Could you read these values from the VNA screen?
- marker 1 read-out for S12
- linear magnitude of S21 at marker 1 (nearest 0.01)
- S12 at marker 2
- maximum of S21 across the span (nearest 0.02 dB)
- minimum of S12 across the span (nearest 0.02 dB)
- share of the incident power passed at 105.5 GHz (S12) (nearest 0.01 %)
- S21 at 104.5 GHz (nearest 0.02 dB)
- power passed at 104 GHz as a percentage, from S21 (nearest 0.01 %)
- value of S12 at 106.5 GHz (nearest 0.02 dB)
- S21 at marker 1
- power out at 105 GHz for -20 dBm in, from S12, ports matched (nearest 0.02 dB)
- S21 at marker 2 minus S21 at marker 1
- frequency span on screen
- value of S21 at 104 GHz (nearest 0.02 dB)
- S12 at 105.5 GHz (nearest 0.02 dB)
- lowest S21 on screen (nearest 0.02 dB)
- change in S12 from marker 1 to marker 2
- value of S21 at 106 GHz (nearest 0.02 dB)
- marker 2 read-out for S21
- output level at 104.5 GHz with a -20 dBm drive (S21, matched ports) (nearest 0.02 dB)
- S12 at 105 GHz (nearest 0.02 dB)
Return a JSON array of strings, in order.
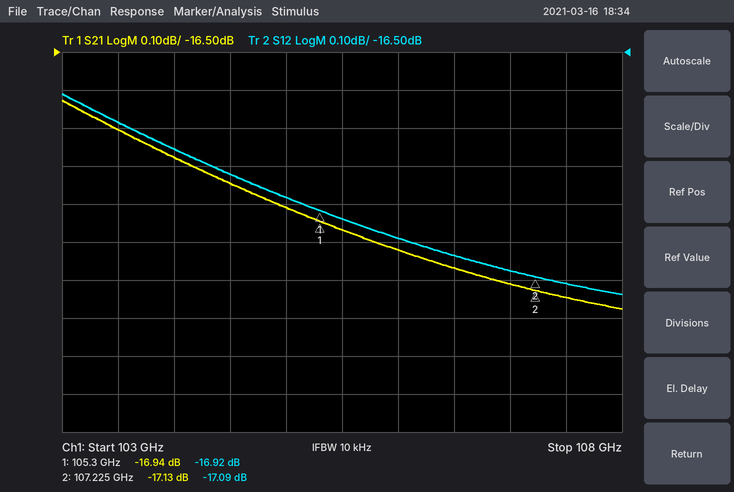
["-16.92 dB", "0.14", "-17.09 dB", "-16.62 dB", "-17.14 dB", "2.02 %", "-16.84 dB", "2.10 %", "-17.04 dB", "-16.94 dB", "-36.88 dBm", "-0.19 dB", "5 GHz", "-16.78 dB", "-16.94 dB", "-17.18 dB", "-0.17 dB", "-17.02 dB", "-17.13 dB", "-36.84 dBm", "-16.88 dB"]
